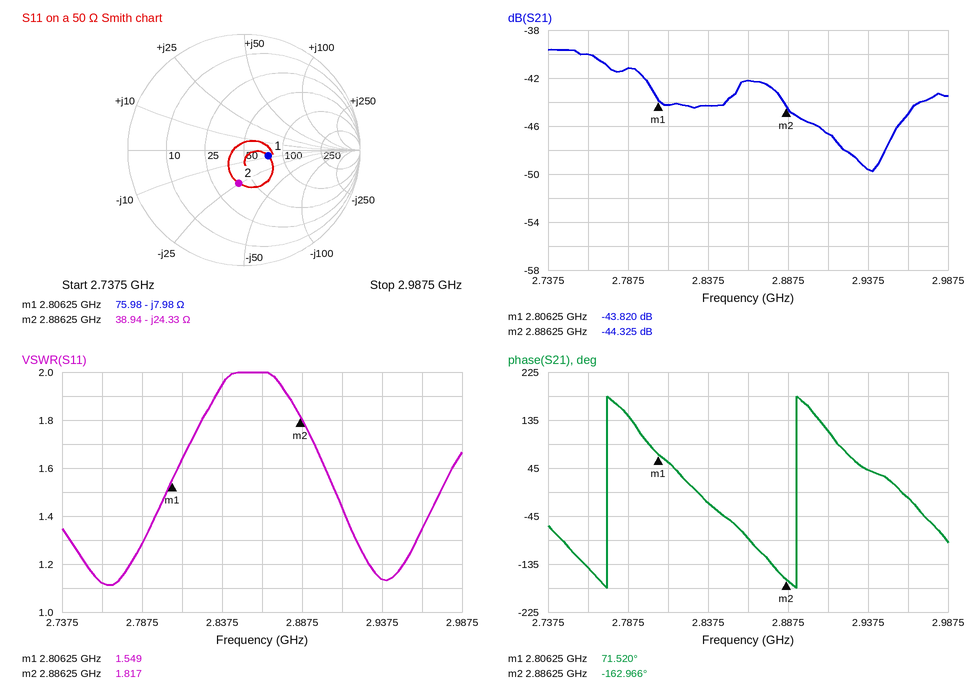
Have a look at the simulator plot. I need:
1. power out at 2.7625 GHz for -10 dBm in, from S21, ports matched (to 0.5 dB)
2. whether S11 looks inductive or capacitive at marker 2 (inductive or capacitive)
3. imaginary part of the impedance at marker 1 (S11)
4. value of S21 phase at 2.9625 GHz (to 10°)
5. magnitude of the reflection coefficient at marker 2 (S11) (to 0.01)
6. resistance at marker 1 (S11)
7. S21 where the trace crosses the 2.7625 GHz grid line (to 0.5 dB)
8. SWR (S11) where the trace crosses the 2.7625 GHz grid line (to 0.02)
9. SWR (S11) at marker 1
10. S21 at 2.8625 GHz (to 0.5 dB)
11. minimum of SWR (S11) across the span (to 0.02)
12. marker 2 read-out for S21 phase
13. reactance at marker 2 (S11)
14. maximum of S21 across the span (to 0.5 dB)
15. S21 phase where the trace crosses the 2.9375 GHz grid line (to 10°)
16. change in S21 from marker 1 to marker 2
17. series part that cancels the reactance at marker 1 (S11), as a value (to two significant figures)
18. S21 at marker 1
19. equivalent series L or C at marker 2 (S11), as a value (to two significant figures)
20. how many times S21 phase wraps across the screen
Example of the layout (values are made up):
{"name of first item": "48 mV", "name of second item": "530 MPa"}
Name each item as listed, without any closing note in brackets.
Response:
{"power out at 2.7625 GHz for -10 dBm in, from S21, ports matched": "-50.0 dBm", "whether S11 looks inductive or capacitive at marker 2": "capacitive", "imaginary part of the impedance at marker 1": "-7.98 Ω", "value of S21 phase at 2.9625 GHz": "-10°", "magnitude of the reflection coefficient at marker 2 (S11)": "0.29", "resistance at marker 1": "75.98 Ω", "S21 where the trace crosses the 2.7625 GHz grid line": "-40.0 dB", "SWR (S11) where the trace crosses the 2.7625 GHz grid line": "1.12", "SWR (S11) at marker 1": "1.549", "S21 at 2.8625 GHz": "-42.0 dB", "minimum of SWR (S11) across the span": "1.12", "marker 2 read-out for S21 phase": "-162.966°", "reactance at marker 2": "-24.33 Ω", "maximum of S21 across the span": "-39.5 dB", "S21 phase where the trace crosses the 2.9375 GHz grid line": "40°", "change in S21 from marker 1 to marker 2": "-0.505 dB", "series part that cancels the reactance at marker 1 (S11), as a value": "450 pH", "S21 at marker 1": "-43.820 dB", "equivalent series L or C at marker 2 (S11), as a value": "2.3 pF", "how many times S21 phase wraps across the screen": "2"}
